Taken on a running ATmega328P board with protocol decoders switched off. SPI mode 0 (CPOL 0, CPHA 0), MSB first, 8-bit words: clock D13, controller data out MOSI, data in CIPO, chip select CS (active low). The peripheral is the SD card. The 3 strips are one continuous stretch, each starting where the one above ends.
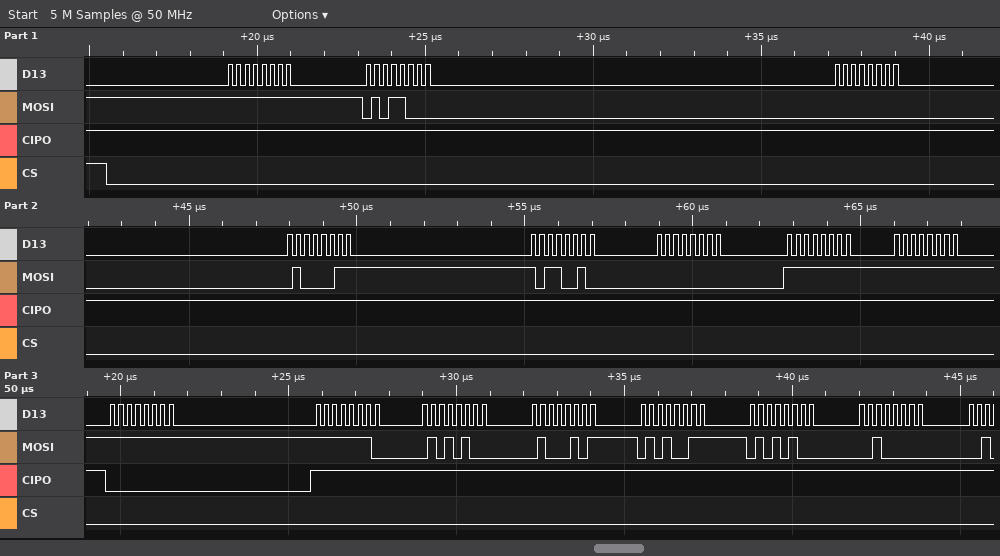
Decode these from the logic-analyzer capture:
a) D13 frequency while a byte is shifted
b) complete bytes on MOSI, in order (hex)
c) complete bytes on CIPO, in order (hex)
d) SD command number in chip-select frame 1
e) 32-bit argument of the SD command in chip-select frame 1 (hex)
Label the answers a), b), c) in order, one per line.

a) 4 MHz
b) FF 58 00 43 B2 00 FF FF FF FE 54 45 53 54 20
c) FF FF FF FF FF FF FF FF 00 FF FF FF FF FF FF
d) CMD24
e) 0x0043B200
